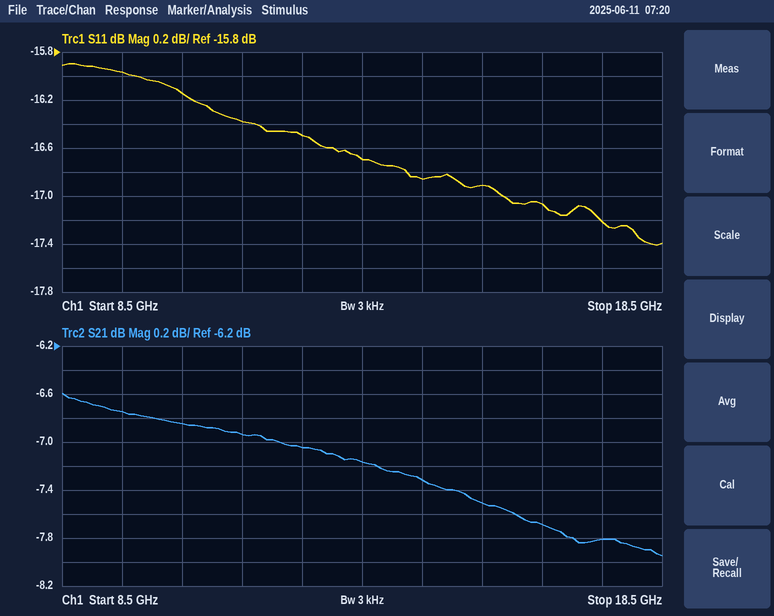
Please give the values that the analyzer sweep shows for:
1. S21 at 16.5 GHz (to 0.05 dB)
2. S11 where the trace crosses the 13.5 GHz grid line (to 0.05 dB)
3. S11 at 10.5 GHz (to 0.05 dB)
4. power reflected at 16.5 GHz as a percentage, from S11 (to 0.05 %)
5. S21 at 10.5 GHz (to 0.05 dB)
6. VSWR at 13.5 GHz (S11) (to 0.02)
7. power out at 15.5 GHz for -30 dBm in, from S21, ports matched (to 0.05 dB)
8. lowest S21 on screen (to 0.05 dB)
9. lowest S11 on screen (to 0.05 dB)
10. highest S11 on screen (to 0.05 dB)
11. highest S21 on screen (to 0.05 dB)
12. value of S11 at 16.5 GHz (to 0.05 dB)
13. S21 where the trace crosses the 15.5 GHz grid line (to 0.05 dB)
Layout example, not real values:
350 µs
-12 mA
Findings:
-7.70 dB
-16.70 dB
-16.15 dB
1.95 %
-6.85 dB
1.34
-37.50 dBm
-7.95 dB
-17.40 dB
-15.90 dB
-6.60 dB
-17.05 dB
-7.50 dB
